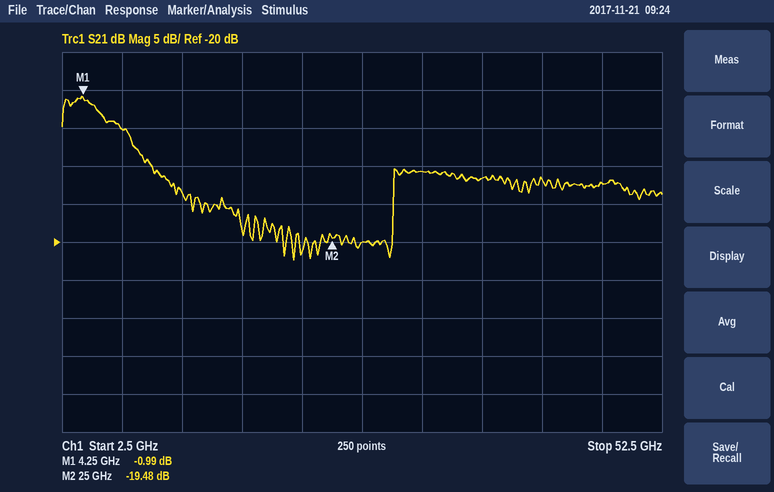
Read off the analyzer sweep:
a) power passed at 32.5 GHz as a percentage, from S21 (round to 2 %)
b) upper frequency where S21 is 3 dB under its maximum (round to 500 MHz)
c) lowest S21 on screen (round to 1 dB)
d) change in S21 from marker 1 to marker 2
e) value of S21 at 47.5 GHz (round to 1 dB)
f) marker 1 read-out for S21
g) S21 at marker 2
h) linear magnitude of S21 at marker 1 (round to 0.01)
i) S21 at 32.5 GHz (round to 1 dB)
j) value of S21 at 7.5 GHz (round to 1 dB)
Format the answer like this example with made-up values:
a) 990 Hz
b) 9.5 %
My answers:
a) 8 %
b) 6.0 GHz
c) -22 dB
d) -18.49 dB
e) -12 dB
f) -0.99 dB
g) -19.48 dB
h) 0.89
i) -11 dB
j) -5 dB
